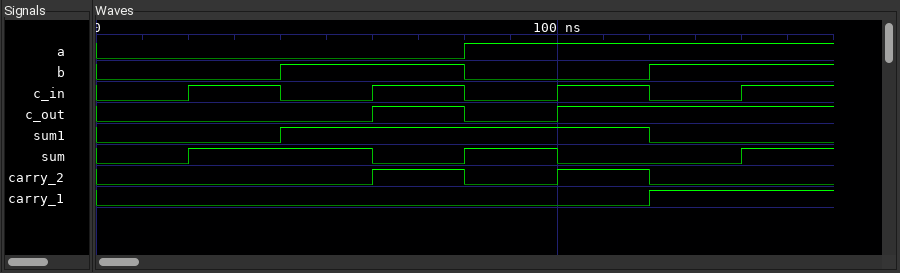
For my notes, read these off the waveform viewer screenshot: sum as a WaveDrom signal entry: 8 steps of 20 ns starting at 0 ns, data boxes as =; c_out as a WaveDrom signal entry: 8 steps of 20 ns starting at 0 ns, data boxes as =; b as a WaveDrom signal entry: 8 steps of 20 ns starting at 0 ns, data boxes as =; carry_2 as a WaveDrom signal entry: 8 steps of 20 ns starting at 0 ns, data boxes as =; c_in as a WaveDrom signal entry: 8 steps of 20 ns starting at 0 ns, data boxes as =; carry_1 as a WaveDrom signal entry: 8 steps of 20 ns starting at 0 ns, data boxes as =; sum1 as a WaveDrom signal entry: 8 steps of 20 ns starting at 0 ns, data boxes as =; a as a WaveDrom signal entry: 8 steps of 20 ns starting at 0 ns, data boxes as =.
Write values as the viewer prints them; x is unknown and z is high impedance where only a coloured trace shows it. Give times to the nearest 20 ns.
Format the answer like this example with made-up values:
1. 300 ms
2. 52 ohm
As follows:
1. {name: 'sum', wave: '01.010.1'}
2. {name: 'c_out', wave: '0..101..'}
3. {name: 'b', wave: '0.1.0.1.'}
4. {name: 'carry_2', wave: '0..1010.'}
5. {name: 'c_in', wave: '01010101'}
6. {name: 'carry_1', wave: '0.....1.'}
7. {name: 'sum1', wave: '0.1...0.'}
8. {name: 'a', wave: '0...1...'}
